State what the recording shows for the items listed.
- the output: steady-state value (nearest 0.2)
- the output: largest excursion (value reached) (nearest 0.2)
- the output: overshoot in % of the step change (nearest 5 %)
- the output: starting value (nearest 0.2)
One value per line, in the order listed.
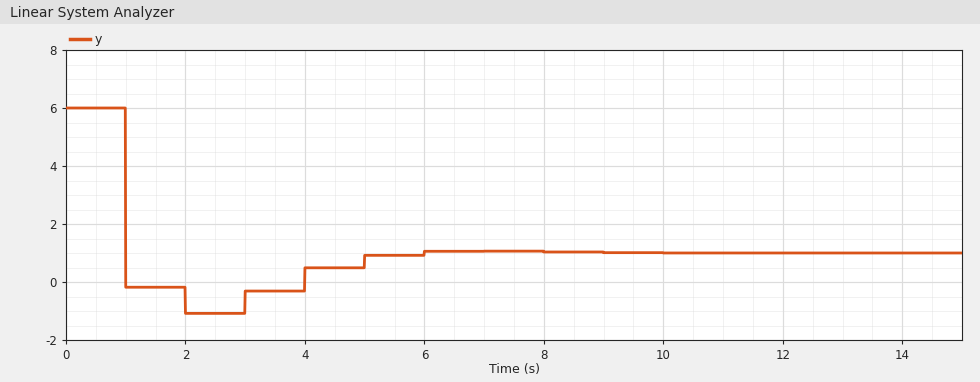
1.0
-1.0
40 %
6.0
